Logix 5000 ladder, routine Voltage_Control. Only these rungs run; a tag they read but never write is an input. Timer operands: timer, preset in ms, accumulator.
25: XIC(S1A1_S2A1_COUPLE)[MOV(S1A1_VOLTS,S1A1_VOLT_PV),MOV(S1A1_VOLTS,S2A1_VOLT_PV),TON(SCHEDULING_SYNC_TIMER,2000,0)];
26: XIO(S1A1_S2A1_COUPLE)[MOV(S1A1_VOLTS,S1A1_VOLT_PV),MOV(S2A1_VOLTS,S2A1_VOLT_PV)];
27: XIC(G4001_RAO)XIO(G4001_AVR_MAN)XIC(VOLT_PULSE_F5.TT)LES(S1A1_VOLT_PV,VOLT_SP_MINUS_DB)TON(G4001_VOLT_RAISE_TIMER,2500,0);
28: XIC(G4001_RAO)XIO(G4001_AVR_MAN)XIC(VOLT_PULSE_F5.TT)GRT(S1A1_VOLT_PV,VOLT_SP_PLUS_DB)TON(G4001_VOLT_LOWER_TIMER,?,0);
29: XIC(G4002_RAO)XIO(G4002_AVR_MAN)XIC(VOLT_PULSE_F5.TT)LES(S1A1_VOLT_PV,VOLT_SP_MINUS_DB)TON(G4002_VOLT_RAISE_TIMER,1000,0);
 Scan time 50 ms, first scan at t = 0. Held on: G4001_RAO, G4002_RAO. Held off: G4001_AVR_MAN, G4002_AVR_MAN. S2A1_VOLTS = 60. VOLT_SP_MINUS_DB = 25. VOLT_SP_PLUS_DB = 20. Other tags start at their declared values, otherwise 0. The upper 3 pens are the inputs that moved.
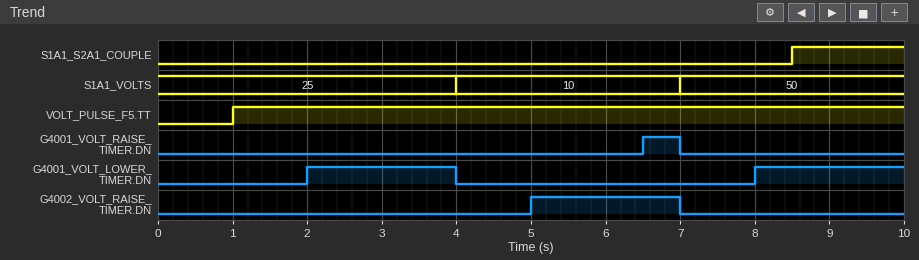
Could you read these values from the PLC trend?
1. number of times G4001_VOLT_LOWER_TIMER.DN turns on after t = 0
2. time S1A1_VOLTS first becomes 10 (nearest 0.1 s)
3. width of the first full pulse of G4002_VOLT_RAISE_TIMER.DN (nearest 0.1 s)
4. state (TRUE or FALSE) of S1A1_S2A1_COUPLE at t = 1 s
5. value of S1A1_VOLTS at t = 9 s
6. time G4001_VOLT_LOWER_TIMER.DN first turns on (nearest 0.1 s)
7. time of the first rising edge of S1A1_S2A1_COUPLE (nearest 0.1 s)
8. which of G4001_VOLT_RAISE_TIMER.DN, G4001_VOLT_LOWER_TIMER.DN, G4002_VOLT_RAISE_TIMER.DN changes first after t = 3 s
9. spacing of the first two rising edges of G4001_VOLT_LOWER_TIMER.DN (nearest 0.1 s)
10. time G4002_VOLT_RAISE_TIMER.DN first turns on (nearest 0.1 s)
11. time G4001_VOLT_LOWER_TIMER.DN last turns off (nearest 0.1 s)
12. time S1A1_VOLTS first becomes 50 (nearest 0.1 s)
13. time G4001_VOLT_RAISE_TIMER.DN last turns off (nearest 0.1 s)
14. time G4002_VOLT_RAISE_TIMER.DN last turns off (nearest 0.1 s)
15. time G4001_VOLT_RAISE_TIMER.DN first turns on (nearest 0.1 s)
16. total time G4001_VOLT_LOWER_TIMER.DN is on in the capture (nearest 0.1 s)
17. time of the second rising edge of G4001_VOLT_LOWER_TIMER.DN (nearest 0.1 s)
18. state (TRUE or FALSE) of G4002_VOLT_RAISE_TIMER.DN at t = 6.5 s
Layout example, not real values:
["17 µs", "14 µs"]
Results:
["2", "4.0 s", "2.0 s", "FALSE", "50", "2.0 s", "8.5 s", "G4001_VOLT_LOWER_TIMER.DN", "6.0 s", "5.0 s", "4.0 s", "7.0 s", "7.0 s", "7.0 s", "6.5 s", "4.0 s", "8.0 s", "TRUE"]
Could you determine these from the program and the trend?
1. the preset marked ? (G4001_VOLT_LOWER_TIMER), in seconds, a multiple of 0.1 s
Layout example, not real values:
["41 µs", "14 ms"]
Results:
["1.0 s"]
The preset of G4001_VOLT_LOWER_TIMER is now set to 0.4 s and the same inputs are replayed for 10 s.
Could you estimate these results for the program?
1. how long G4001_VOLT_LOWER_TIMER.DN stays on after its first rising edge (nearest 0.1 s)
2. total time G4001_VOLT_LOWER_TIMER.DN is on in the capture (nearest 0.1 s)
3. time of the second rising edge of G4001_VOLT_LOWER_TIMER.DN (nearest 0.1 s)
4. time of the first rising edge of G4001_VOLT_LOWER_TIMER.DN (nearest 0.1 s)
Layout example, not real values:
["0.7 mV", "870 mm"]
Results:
["2.6 s", "5.2 s", "7.4 s", "1.4 s"]
